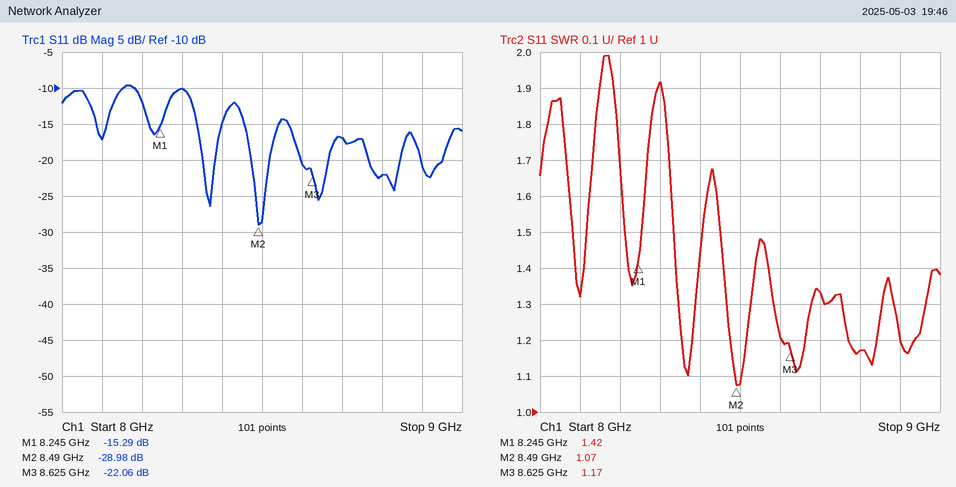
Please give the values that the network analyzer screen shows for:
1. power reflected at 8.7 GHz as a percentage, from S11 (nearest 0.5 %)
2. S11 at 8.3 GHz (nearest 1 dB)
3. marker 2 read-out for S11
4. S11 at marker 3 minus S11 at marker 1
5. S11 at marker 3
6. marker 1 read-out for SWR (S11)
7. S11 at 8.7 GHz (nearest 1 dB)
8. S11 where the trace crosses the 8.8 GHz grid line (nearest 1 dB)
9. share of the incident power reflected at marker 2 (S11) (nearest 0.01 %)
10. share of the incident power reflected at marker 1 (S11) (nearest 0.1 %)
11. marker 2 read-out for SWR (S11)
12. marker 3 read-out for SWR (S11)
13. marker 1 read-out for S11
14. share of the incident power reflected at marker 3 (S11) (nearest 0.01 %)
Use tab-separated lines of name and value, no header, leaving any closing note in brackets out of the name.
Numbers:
power reflected at 8.7 GHz as a percentage, from S11	2.0 %
S11 at 8.3 GHz	-10 dB
marker 2 read-out for S11	-28.98 dB
S11 at marker 3 minus S11 at marker 1	-6.77 dB
S11 at marker 3	-22.06 dB
marker 1 read-out for SWR	1.42
S11 at 8.7 GHz	-17 dB
S11 where the trace crosses the 8.8 GHz grid line	-22 dB
share of the incident power reflected at marker 2 (S11)	0.13 %
share of the incident power reflected at marker 1 (S11)	3.0 %
marker 2 read-out for SWR	1.07
marker 3 read-out for SWR	1.17
marker 1 read-out for S11	-15.29 dB
share of the incident power reflected at marker 3 (S11)	0.62 %
